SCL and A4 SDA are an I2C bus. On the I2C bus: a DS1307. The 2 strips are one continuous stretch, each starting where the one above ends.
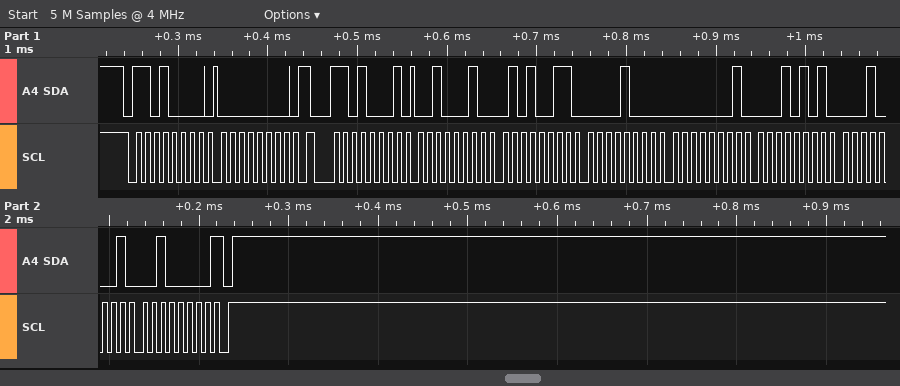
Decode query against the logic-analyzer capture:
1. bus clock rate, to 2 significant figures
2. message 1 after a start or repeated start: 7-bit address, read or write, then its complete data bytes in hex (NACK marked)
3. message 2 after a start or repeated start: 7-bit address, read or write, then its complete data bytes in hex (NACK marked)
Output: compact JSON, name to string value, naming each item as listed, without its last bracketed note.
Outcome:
{"bus clock rate, to 2 significant figures": "100 kHz", "message 1 after a start or repeated start: 7-bit address, read or write, then its complete data bytes in hex": "0x68 write: 00", "message 2 after a start or repeated start: 7-bit address, read or write, then its complete data bytes in hex": "0x68 read: 22 53 08 01 15 11 20 NACK"}
